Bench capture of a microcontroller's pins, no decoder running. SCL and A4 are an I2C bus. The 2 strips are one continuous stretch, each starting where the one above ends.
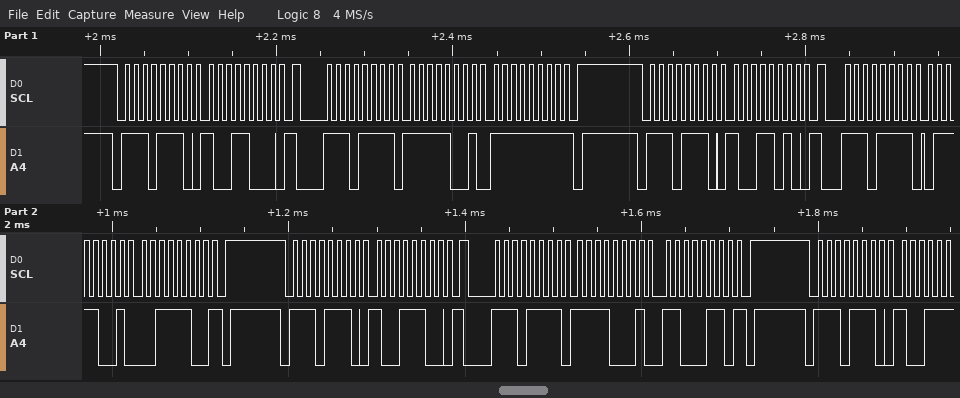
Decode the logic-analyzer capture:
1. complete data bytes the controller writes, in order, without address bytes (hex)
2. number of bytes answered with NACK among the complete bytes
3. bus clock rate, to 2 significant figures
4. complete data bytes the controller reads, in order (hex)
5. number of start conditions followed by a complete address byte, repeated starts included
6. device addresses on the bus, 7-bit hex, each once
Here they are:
98 9A 9C
3
100 kHz
F9 FF 79 3C F1 C6
7
0x77
